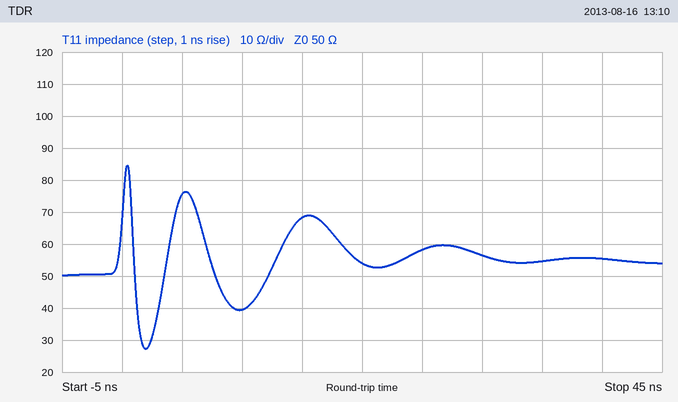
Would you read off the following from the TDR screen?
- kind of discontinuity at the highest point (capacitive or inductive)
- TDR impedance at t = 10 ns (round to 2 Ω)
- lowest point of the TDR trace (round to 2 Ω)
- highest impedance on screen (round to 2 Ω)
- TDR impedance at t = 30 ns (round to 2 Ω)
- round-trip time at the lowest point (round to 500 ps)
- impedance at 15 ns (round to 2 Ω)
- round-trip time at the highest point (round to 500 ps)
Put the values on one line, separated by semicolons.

inductive; 40 Ω; 28 Ω; 84 Ω; 56 Ω; 2.0 ns; 68 Ω; 500 ps
